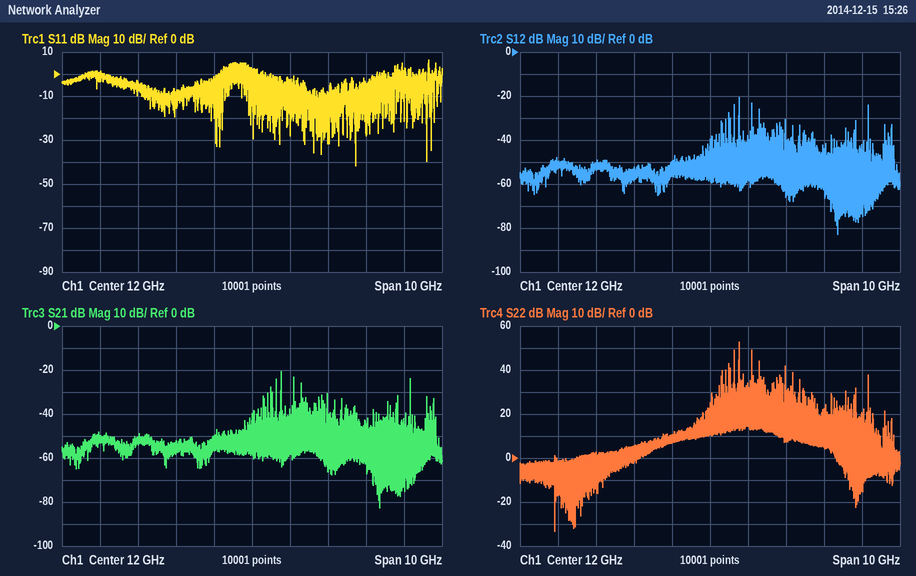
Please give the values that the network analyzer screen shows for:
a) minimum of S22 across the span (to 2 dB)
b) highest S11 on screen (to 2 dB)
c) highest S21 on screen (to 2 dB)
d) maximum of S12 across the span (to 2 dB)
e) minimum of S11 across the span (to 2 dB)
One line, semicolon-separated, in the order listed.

-34 dB; 6 dB; -20 dB; -20 dB; -42 dB
